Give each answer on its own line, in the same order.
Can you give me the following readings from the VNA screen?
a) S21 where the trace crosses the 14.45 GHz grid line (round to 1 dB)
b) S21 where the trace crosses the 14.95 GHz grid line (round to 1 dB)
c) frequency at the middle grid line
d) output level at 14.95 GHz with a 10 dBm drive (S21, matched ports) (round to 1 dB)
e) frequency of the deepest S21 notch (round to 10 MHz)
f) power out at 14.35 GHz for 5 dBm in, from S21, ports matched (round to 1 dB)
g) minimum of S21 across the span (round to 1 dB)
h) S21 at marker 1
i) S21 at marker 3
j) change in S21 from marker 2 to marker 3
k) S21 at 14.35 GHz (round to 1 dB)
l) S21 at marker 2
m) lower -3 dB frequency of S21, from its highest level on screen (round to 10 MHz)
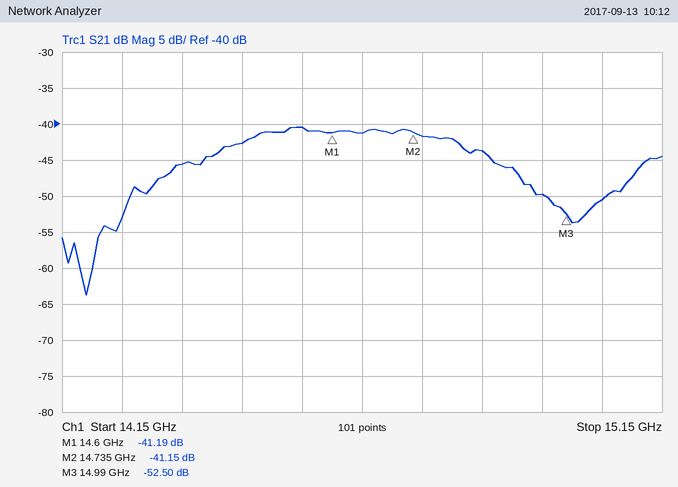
-43 dB
-50 dB
14.65 GHz
-40 dBm
14.19 GHz
-41 dBm
-64 dB
-41.19 dB
-52.50 dB
-11.35 dB
-46 dB
-41.15 dB
14.42 GHz
